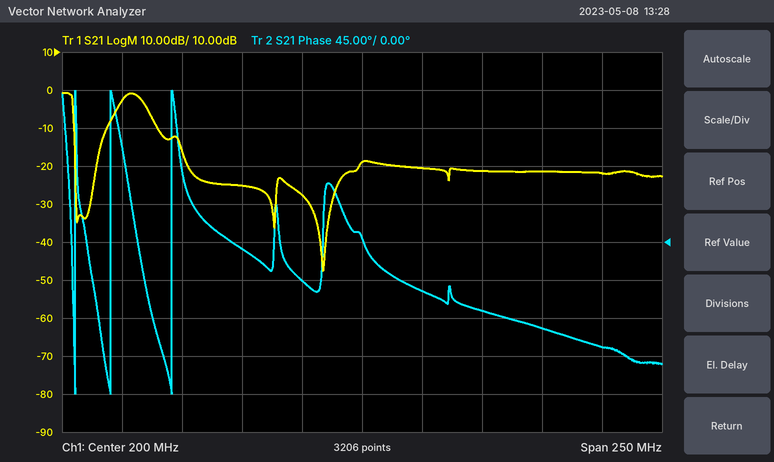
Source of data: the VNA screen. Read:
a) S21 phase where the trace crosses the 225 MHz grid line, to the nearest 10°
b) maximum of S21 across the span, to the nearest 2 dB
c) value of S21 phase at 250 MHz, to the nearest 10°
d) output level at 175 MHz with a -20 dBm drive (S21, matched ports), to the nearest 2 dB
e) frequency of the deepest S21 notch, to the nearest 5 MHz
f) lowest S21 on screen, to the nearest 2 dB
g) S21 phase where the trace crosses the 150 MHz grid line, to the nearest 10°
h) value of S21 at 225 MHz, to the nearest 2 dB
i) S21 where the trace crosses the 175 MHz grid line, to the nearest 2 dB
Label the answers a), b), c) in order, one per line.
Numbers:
a) -60°
b) 0 dB
c) -80°
d) -48 dBm
e) 185 MHz
f) -48 dB
g) -10°
h) -20 dB
i) -28 dB
